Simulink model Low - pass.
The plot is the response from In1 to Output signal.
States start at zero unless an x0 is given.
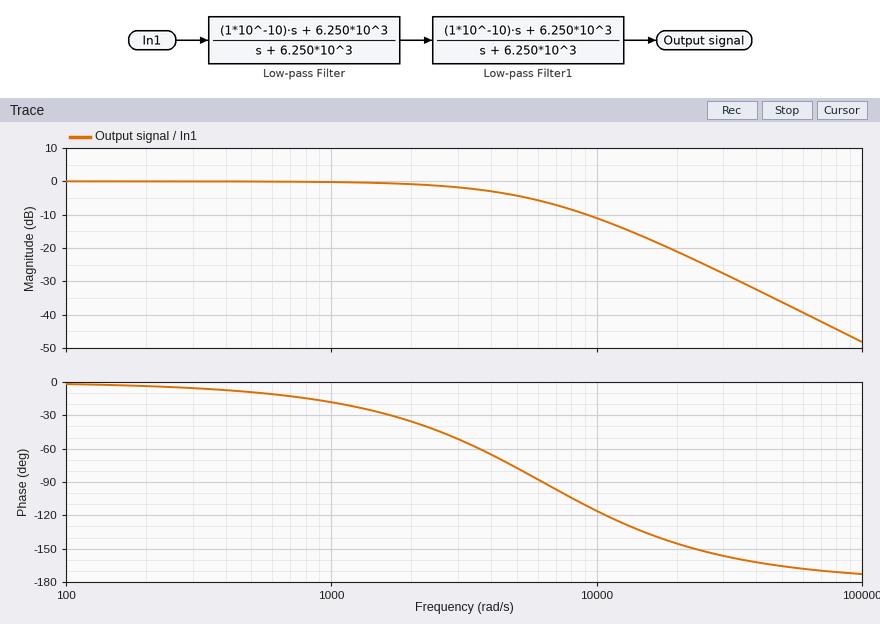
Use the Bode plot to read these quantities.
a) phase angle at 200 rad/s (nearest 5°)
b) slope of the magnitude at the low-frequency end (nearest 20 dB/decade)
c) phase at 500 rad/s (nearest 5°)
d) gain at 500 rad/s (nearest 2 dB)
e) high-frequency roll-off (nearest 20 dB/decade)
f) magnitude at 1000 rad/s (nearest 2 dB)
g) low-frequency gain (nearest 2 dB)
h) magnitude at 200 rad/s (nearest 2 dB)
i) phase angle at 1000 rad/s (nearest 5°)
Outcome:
-5°
0 dB/decade
-10°
0 dB
-40 dB/decade
0 dB
0 dB
0 dB
-20°
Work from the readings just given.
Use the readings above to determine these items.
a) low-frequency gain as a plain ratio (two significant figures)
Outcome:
1.0
